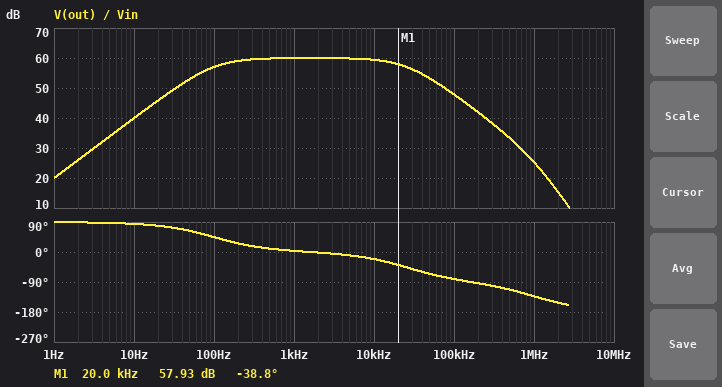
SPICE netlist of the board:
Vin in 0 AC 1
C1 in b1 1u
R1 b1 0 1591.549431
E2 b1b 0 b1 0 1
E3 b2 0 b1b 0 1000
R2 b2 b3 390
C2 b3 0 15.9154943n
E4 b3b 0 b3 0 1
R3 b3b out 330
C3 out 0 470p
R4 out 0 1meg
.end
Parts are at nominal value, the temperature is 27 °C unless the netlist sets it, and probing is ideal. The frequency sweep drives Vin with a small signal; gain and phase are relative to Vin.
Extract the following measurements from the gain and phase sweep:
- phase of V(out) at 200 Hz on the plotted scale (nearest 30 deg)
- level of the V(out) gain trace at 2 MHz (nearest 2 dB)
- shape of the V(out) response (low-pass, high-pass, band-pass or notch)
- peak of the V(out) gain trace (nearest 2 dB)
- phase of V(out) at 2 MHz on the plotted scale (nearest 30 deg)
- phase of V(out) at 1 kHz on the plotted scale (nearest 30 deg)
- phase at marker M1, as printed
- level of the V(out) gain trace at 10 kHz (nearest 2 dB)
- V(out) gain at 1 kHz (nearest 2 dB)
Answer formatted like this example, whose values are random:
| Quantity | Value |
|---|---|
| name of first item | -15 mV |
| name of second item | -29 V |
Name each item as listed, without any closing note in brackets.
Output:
| Quantity | Value |
|---|---|
| phase of V(out) at 200 Hz on the plotted scale | 30 deg |
| level of the V(out) gain trace at 2 MHz | 16 dB |
| shape of the V(out) response | band-pass |
| peak of the V(out) gain trace | 60 dB |
| phase of V(out) at 2 MHz on the plotted scale | -150 deg |
| phase of V(out) at 1 kHz on the plotted scale | 0 deg |
| phase at marker M1, as printed | -38.8 deg |
| level of the V(out) gain trace at 10 kHz | 60 dB |
| V(out) gain at 1 kHz | 60 dB |
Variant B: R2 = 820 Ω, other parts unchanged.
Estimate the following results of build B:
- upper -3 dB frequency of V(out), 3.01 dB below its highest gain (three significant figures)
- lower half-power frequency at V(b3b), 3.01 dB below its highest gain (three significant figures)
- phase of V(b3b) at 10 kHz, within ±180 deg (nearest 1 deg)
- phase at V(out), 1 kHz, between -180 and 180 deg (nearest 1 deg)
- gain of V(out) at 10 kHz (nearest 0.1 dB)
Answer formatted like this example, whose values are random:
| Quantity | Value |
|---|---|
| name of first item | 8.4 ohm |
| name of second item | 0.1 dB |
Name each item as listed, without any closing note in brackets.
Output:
| Quantity | Value |
|---|---|
| upper -3 dB frequency of V(out), 3.01 dB below its highest gain | 12.4 kHz |
| lower half-power frequency at V(b3b), 3.01 dB below its highest gain | 98.4 Hz |
| phase of V(b3b) at 10 kHz, within ±180 deg | -39 deg |
| phase at V(out), 1 kHz, between -180 and 180 deg | 1 deg |
| gain of V(out) at 10 kHz | 57.8 dB |
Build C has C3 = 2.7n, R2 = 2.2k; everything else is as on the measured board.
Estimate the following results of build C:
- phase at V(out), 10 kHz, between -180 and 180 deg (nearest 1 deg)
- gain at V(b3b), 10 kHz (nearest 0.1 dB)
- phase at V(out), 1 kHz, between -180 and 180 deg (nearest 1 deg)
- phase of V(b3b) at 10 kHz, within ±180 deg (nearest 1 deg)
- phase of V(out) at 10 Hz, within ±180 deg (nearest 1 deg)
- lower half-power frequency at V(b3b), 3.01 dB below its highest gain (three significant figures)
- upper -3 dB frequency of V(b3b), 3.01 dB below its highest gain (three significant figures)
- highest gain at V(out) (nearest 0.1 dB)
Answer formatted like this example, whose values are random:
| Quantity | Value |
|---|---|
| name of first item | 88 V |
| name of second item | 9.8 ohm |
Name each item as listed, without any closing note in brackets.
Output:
| Quantity | Value |
|---|---|
| phase at V(out), 10 kHz, between -180 and 180 deg | -68 deg |
| gain at V(b3b), 10 kHz | 52.3 dB |
| phase at V(out), 1 kHz, between -180 and 180 deg | -7 deg |
| phase of V(b3b) at 10 kHz, within ±180 deg | -65 deg |
| phase of V(out) at 10 Hz, within ±180 deg | 84 deg |
| lower half-power frequency at V(b3b), 3.01 dB below its highest gain | 95.9 Hz |
| upper -3 dB frequency of V(b3b), 3.01 dB below its highest gain | 4.74 kHz |
| highest gain at V(out) | 59.8 dB |
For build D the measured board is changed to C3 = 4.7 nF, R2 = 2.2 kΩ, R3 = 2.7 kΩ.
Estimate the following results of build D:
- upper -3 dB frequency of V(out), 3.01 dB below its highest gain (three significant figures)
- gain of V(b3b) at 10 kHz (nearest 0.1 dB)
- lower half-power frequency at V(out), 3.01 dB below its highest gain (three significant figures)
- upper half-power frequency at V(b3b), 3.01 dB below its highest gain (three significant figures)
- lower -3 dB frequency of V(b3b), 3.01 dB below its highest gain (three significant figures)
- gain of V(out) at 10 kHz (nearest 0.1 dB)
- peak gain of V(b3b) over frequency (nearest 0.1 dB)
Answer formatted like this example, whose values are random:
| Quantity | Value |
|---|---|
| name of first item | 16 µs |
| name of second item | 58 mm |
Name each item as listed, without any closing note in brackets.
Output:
| Quantity | Value |
|---|---|
| upper -3 dB frequency of V(out), 3.01 dB below its highest gain | 4.26 kHz |
| gain of V(b3b) at 10 kHz | 52.3 dB |
| lower half-power frequency at V(out), 3.01 dB below its highest gain | 95.6 Hz |
| upper half-power frequency at V(b3b), 3.01 dB below its highest gain | 4.74 kHz |
| lower -3 dB frequency of V(b3b), 3.01 dB below its highest gain | 95.9 Hz |
| gain of V(out) at 10 kHz | 50.2 dB |
| peak gain of V(b3b) over frequency | 59.8 dB |
